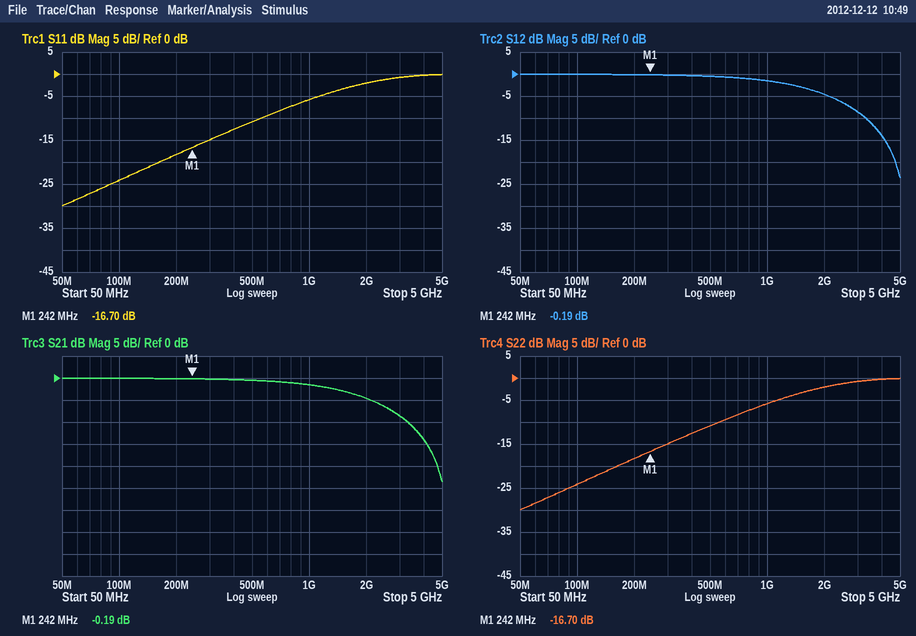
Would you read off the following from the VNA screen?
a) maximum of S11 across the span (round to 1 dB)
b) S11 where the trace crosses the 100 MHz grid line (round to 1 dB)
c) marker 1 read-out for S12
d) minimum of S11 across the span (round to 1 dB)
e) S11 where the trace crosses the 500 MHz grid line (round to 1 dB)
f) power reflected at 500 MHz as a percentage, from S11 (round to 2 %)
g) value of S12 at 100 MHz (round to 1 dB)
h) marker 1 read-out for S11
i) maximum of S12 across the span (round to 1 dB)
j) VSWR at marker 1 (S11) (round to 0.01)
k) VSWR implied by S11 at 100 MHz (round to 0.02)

0 dB
-24 dB
-0.19 dB
-30 dB
-11 dB
8 %
0 dB
-16.70 dB
0 dB
1.34
1.14
